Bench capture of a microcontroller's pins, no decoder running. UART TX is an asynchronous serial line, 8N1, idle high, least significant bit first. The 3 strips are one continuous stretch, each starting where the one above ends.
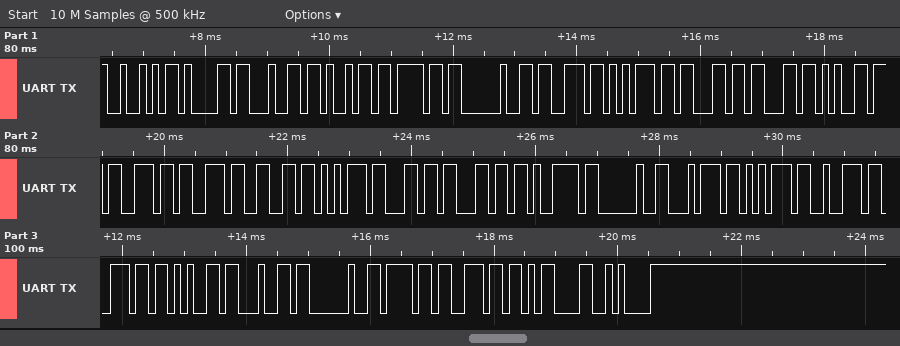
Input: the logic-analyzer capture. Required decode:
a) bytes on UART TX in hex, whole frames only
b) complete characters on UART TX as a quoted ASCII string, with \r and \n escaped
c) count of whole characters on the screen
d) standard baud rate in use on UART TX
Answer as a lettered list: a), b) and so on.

a) 52 61 64 69 6F 20 73 75 63 63 65 73 73 66 75 6C 6C 79 20 74 75 72 6E 65 64 20 6F 6E 0D 0A
b) "Radio successfully turned on\r\n"
c) 30
d) 9600 baud
